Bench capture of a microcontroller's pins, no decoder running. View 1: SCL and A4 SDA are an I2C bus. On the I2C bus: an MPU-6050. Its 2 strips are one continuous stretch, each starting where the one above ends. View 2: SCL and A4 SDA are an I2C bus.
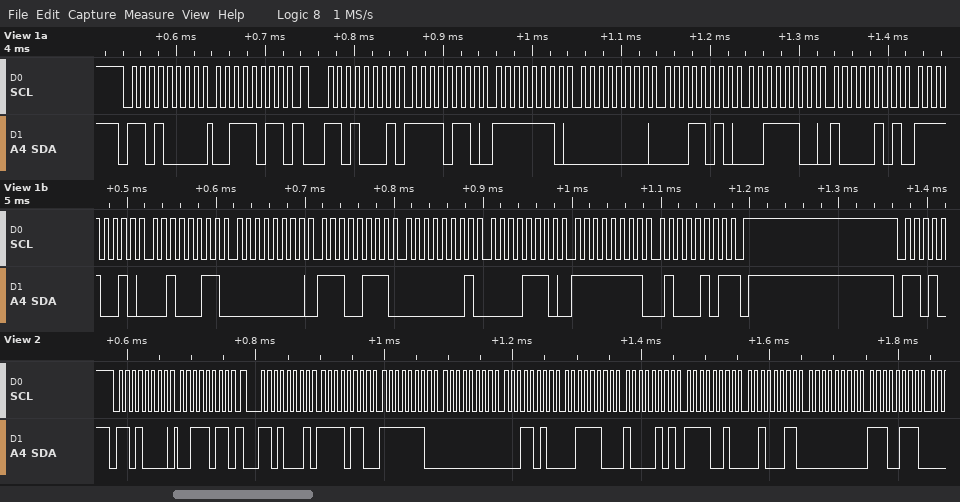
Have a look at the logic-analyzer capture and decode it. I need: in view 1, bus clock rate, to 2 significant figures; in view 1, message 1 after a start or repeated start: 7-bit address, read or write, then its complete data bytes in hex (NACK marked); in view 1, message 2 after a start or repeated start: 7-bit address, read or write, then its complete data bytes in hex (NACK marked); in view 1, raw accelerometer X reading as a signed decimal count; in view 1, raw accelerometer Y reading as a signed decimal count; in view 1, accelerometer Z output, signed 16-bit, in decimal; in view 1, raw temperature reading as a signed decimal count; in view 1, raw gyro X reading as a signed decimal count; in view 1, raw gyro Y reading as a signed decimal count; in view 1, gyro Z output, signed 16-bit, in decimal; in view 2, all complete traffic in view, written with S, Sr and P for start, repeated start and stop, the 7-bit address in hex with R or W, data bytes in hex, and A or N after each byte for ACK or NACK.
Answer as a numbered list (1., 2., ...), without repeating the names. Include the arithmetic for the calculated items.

1. 100 kHz
2. 0x68 write: 3B
3. 0x68 read: F6 FE 00 1A 3C 85 F2 23 00 E7 01 0E FF 45 NACK
4. 0xF6FE = -2306
5. 0x001A = 26
6. 0x3C85 = 15493
7. 0xF223 = -3549
8. 0x00E7 = 231
9. 0x010E = 270
10. 0xFF45 = -187
11. S 68W A 3B A Sr 68R A F6 A FE A 00 A 1A A 3C A 85 A F2 A 23 A 00 A E7 A
